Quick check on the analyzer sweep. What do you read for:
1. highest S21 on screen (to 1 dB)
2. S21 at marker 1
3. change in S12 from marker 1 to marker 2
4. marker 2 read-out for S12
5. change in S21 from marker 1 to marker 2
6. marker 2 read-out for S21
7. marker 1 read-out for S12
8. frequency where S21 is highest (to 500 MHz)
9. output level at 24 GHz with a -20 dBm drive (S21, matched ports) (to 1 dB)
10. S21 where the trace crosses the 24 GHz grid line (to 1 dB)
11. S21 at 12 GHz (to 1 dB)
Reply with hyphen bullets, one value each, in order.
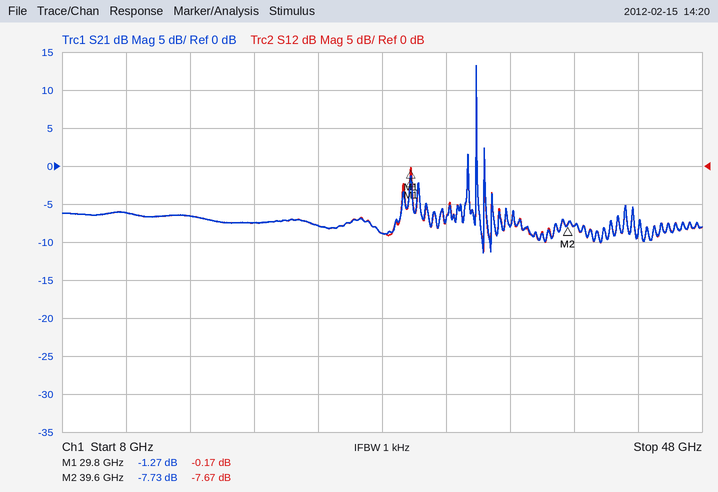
- 13 dB
- -1.27 dB
- -7.50 dB
- -7.67 dB
- -6.46 dB
- -7.73 dB
- -0.17 dB
- 34.0 GHz
- -28 dBm
- -8 dB
- -6 dB
